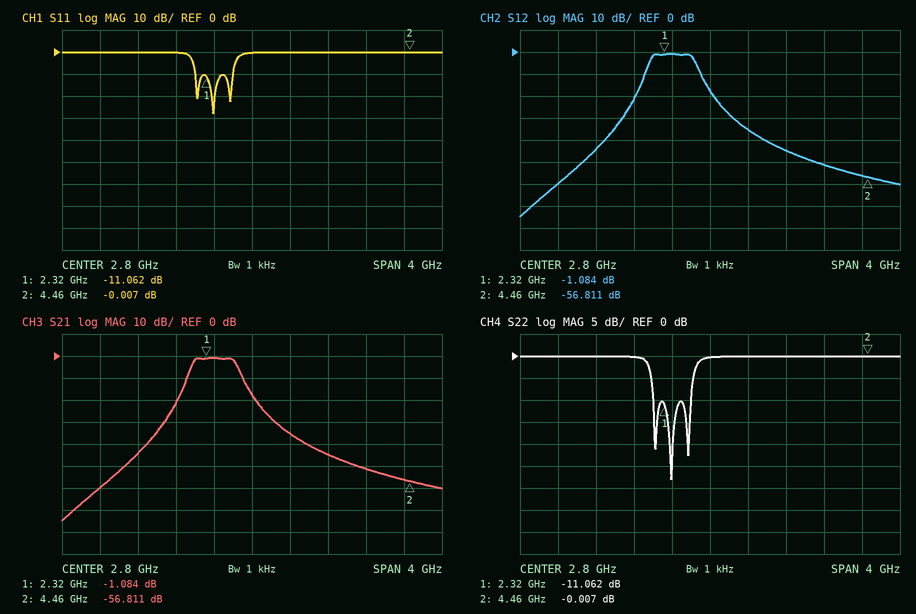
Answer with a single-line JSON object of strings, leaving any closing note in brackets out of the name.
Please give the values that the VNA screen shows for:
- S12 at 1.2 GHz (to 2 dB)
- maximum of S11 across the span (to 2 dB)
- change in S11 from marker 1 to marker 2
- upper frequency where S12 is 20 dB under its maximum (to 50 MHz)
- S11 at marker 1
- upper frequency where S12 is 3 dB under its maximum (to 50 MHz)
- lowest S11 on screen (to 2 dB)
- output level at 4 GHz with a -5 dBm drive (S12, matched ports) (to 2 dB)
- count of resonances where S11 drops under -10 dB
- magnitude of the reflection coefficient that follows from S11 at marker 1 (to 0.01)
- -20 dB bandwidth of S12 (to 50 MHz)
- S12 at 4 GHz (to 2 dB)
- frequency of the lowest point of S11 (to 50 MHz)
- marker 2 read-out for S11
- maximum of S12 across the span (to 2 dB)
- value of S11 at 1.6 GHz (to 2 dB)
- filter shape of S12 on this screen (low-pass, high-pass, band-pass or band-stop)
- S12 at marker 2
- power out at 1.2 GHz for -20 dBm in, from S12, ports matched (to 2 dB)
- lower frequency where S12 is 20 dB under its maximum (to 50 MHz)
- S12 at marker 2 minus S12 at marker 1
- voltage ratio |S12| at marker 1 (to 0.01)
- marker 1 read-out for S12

{"S12 at 1.2 GHz": "-60 dB", "maximum of S11 across the span": "0 dB", "change in S11 from marker 1 to marker 2": "11.055 dB", "upper frequency where S12 is 20 dB under its maximum": "2.85 GHz", "S11 at marker 1": "-11.062 dB", "upper frequency where S12 is 3 dB under its maximum": "2.65 GHz", "lowest S11 on screen": "-28 dB", "output level at 4 GHz with a -5 dBm drive (S12, matched ports)": "-56 dBm", "count of resonances where S11 drops under -10 dB": "3", "magnitude of the reflection coefficient that follows from S11 at marker 1": "0.28", "-20 dB bandwidth of S12": "850 MHz", "S12 at 4 GHz": "-52 dB", "frequency of the lowest point of S11": "2.40 GHz", "marker 2 read-out for S11": "-0.007 dB", "maximum of S12 across the span": "0 dB", "value of S11 at 1.6 GHz": "0 dB", "filter shape of S12 on this screen": "band-pass", "S12 at marker 2": "-56.811 dB", "power out at 1.2 GHz for -20 dBm in, from S12, ports matched": "-80 dBm", "lower frequency where S12 is 20 dB under its maximum": "2.00 GHz", "S12 at marker 2 minus S12 at marker 1": "-55.727 dB", "voltage ratio |S12| at marker 1": "0.88", "marker 1 read-out for S12": "-1.084 dB"}
